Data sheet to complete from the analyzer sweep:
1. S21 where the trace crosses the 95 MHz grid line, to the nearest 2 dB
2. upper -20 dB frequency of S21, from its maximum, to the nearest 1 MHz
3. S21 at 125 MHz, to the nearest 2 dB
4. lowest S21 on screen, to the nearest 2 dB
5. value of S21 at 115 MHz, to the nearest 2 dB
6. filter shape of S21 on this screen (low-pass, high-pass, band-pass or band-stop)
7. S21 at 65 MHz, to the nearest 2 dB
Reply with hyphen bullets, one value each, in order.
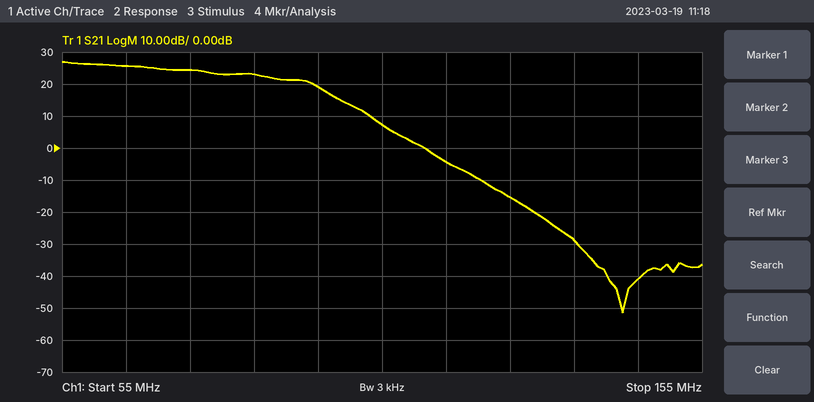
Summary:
- 20 dB
- 105 MHz
- -16 dB
- -52 dB
- -4 dB
- low-pass
- 26 dB
